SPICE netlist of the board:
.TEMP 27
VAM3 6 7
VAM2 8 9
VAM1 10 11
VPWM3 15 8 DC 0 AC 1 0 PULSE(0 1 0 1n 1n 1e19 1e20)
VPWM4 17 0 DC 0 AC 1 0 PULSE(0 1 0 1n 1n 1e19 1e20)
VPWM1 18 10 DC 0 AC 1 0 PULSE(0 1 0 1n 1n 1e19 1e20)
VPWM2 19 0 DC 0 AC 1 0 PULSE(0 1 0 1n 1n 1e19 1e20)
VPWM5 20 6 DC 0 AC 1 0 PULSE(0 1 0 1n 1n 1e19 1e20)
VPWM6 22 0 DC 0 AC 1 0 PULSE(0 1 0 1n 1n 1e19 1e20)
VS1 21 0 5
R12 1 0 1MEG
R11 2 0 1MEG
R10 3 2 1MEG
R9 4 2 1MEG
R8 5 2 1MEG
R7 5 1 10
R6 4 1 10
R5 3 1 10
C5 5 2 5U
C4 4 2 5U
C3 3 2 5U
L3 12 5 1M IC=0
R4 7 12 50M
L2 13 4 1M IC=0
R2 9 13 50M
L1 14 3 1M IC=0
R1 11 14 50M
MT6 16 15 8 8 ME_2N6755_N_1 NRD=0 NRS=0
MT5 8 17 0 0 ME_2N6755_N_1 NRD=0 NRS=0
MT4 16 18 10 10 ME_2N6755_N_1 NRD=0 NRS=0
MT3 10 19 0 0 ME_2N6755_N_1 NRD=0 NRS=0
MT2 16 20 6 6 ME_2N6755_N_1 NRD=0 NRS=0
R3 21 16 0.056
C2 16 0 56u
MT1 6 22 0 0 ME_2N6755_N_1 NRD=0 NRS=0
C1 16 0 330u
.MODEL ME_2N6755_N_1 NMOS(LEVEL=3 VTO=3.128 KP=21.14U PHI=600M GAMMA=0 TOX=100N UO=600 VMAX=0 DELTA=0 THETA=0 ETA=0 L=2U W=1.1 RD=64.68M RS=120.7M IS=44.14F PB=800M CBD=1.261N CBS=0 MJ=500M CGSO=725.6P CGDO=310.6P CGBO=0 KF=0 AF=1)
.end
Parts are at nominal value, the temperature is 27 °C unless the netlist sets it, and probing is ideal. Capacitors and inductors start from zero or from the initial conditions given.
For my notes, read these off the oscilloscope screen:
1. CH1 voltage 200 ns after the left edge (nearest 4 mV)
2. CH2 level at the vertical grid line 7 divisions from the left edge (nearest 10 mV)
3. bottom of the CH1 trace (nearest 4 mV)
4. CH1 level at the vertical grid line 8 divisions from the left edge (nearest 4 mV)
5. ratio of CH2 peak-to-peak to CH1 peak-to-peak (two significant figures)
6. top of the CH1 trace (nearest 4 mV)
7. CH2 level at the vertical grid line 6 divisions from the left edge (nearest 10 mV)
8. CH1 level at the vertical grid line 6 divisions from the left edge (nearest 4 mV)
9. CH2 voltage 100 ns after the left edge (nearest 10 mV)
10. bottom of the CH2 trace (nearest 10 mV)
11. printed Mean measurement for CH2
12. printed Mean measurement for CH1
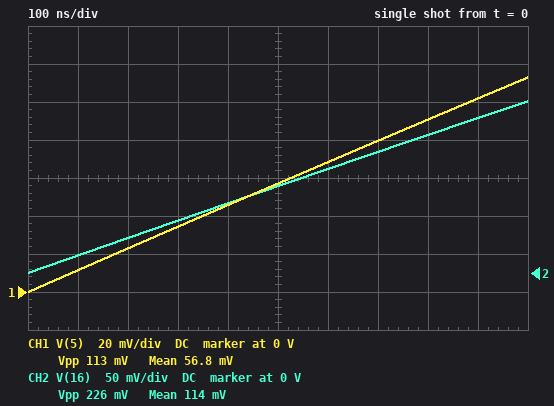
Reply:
24 mV
160 mV
0 V
92 mV
2.0
112 mV
140 mV
68 mV
20 mV
0 V
114 mV
56.8 mV
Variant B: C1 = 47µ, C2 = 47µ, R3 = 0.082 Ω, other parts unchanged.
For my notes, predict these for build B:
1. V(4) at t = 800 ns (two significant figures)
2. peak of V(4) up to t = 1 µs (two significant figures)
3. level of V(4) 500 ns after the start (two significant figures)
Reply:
250 mV
300 mV
160 mV
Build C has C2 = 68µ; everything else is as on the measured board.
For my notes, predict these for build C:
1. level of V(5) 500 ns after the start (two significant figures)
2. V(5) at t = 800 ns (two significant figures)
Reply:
55 mV
88 mV
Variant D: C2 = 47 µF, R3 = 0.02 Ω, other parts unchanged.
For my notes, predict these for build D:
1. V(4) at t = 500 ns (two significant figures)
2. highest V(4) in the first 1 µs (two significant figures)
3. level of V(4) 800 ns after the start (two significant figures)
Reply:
160 mV
310 mV
250 mV
